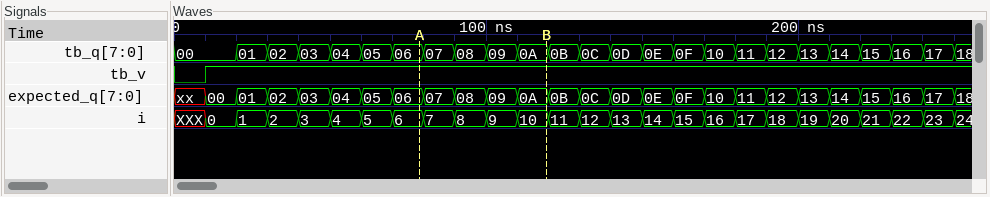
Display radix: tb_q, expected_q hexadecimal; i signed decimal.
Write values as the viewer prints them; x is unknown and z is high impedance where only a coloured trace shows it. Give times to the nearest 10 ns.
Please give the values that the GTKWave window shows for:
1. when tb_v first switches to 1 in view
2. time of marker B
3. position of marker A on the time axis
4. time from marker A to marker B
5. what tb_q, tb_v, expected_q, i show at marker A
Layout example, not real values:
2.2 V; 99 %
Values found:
10 ns; 120 ns; 80 ns; 40 ns; tb_q=06, tb_v=1, expected_q=06, i=6
